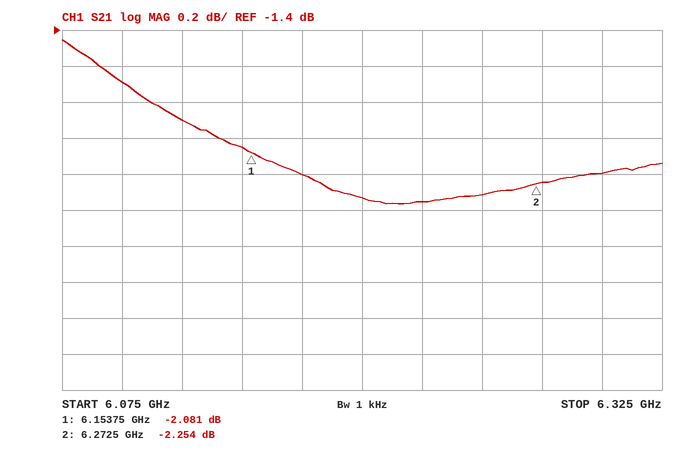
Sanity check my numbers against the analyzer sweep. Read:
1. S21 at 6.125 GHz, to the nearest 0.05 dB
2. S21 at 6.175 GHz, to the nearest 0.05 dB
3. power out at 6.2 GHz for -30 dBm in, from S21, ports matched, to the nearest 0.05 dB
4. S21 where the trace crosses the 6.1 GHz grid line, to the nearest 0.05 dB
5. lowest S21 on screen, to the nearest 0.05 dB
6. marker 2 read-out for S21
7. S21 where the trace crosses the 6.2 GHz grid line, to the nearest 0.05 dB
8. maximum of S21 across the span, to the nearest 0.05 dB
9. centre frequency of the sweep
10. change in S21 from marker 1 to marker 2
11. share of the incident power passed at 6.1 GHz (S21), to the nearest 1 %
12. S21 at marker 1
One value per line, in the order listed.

-1.90 dB
-2.20 dB
-32.35 dBm
-1.70 dB
-2.35 dB
-2.254 dB
-2.35 dB
-1.45 dB
6.2 GHz
-0.173 dB
68 %
-2.081 dB
